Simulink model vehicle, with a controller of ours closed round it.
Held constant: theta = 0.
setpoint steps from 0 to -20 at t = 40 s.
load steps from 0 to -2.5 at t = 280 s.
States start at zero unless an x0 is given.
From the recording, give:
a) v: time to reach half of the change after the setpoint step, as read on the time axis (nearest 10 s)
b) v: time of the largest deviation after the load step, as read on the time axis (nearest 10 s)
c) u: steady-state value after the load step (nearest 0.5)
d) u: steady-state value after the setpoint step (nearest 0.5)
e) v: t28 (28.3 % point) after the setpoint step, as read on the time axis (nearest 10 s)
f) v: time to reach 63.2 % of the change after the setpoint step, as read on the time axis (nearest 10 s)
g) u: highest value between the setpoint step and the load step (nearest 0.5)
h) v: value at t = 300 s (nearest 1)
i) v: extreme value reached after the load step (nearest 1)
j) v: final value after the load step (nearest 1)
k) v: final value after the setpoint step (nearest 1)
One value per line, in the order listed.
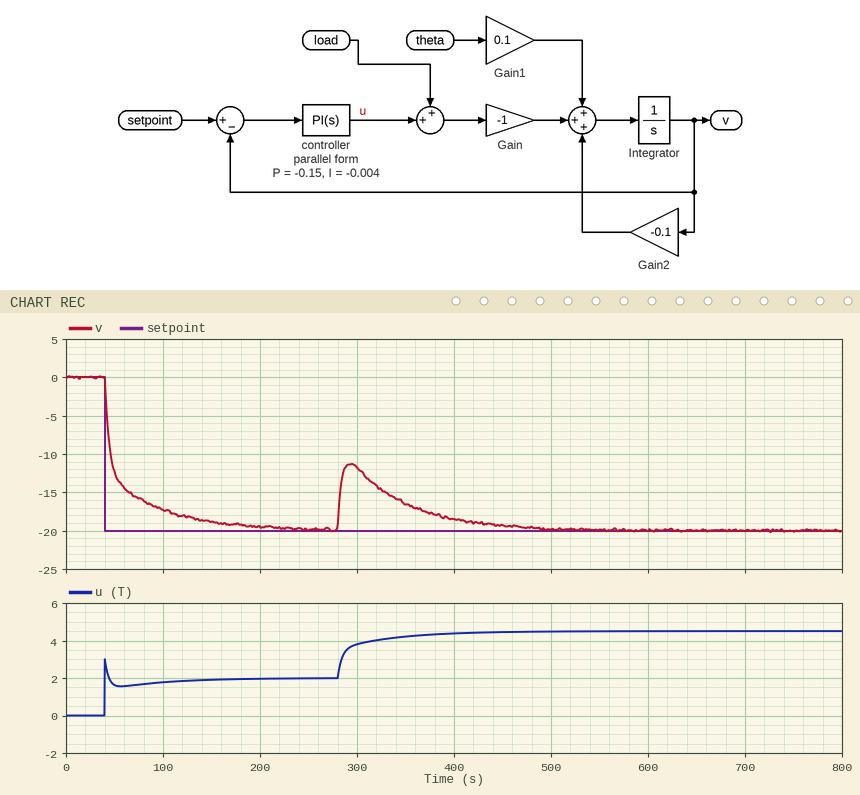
50 s
290 s
4.5
2.0
40 s
50 s
3.0
-12
-11
-20
-20
